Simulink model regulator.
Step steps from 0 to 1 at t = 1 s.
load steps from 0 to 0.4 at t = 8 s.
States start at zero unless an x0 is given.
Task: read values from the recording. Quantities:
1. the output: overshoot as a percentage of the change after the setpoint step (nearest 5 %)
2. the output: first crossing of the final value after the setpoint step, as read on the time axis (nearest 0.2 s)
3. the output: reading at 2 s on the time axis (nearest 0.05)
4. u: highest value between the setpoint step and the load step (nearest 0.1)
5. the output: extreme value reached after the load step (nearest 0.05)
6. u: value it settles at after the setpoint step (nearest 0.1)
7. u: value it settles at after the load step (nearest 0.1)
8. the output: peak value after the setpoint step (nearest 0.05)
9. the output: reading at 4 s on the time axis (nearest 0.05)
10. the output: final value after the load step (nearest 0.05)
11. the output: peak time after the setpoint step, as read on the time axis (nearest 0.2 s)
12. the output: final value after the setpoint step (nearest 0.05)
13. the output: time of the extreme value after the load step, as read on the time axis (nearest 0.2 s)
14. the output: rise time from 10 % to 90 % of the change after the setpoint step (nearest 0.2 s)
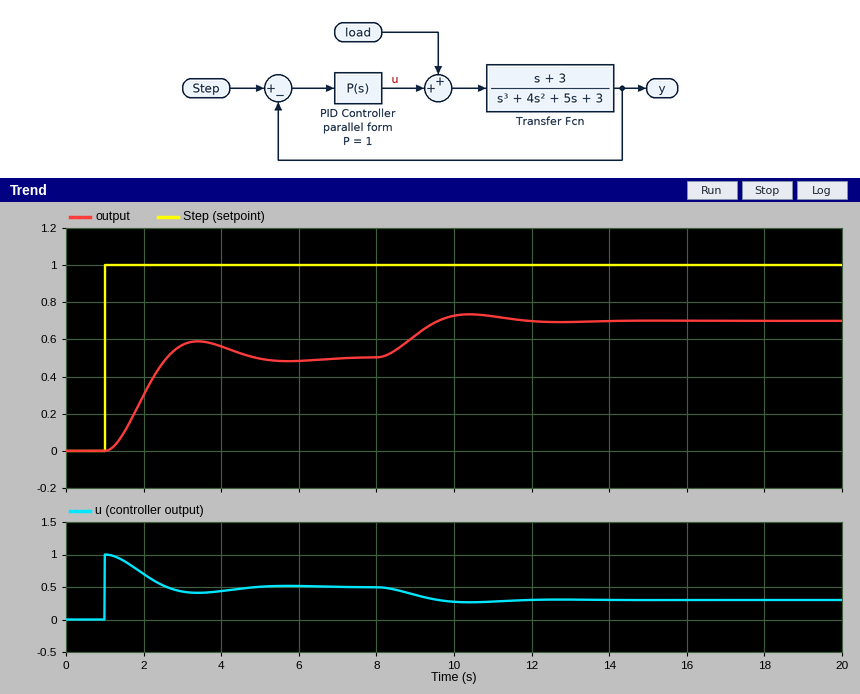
20 %
2.6 s
0.30
1.0
0.75
0.5
0.3
0.60
0.55
0.70
3.4 s
0.50
10.4 s
1.0 s
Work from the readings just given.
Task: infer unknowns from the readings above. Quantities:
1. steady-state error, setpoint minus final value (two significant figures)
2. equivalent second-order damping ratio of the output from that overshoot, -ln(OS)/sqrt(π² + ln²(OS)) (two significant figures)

0.50
0.46
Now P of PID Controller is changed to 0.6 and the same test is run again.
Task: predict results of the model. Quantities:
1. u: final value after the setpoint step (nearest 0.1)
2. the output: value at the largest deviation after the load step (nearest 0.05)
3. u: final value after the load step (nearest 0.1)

0.4
0.65
0.2
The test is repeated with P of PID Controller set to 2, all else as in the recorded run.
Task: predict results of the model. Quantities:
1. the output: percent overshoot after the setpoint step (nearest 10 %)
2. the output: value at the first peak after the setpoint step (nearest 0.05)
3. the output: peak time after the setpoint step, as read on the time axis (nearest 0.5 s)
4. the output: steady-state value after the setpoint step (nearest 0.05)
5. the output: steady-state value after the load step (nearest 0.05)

30 %
0.85
3.0 s
0.65
0.80
